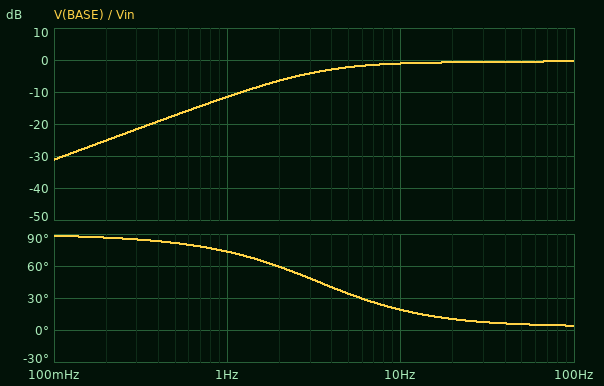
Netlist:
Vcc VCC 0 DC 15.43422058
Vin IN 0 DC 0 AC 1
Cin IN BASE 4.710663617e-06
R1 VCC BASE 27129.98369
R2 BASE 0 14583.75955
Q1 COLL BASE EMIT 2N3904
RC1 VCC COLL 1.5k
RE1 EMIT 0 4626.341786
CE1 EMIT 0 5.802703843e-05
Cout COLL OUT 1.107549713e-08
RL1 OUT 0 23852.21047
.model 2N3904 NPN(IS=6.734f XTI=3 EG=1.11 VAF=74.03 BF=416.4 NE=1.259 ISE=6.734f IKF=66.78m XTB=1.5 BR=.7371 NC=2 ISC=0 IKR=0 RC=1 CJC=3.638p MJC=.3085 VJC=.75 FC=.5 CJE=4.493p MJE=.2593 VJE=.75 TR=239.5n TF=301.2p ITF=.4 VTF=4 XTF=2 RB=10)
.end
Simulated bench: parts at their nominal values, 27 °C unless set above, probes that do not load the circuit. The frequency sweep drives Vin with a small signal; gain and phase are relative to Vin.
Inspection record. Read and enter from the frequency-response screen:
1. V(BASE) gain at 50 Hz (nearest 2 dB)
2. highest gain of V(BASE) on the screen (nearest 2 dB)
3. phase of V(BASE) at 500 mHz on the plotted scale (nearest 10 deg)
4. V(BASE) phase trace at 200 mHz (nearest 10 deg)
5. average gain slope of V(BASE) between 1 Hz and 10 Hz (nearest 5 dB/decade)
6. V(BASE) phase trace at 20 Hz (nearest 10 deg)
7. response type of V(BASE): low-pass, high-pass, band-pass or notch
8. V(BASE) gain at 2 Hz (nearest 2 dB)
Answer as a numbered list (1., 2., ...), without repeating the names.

1. 0 dB
2. 0 dB
3. 80 deg
4. 90 deg
5. 10 dB/decade
6. 10 deg
7. high-pass
8. -6 dB
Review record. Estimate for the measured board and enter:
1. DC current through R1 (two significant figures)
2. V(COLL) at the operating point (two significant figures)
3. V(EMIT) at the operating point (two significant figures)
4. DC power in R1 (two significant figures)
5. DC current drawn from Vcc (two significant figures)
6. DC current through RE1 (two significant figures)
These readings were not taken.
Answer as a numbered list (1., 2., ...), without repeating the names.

1. 370 µA
2. 14 V
3. 4.7 V
4. 3.8 mW
5. 1.4 mA
6. 1.0 mA
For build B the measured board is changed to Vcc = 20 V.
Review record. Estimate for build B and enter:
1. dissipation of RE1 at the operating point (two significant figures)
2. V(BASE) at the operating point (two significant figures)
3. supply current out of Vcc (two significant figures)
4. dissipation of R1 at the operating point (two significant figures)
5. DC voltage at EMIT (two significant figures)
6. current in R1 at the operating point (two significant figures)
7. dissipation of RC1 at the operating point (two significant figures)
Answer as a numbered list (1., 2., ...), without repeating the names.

1. 8.4 mW
2. 6.9 V
3. 1.8 mA
4. 6.3 mW
5. 6.2 V
6. 480 µA
7. 2.7 mW
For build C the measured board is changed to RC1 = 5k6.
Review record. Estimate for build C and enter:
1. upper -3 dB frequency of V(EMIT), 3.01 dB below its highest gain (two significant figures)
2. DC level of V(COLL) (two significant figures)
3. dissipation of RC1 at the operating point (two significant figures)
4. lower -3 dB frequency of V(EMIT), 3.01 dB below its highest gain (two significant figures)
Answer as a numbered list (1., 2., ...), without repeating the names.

1. 110 Hz
2. 9.8 V
3. 5.6 mW
4. 3.1 Hz
